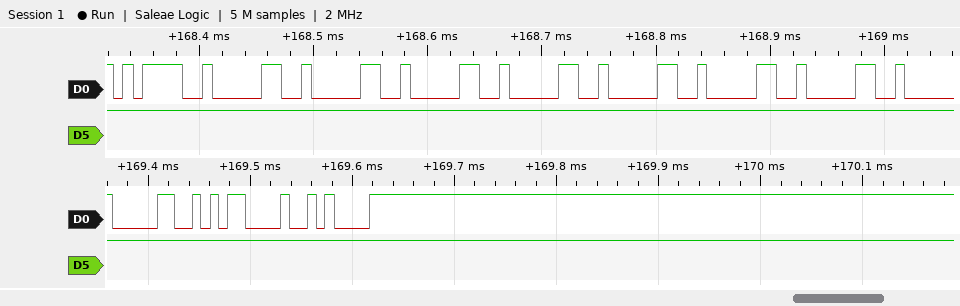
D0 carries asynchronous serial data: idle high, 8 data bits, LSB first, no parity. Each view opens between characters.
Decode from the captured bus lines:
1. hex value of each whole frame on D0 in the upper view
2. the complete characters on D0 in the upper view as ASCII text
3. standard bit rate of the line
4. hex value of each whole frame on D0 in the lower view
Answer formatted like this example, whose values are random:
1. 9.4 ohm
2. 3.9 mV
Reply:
1. 3D, 30, 30, 30, 30, 30, 30, 30
2. "=0000000"
3. 115200 baud
4. 30, 0D, 0A
